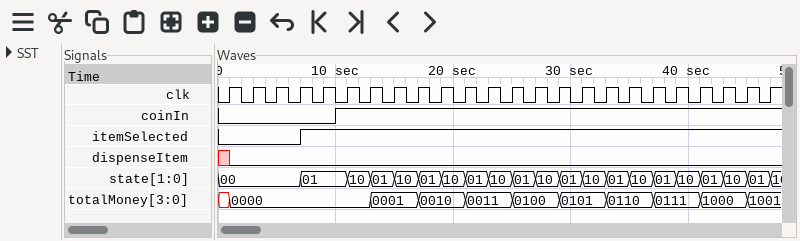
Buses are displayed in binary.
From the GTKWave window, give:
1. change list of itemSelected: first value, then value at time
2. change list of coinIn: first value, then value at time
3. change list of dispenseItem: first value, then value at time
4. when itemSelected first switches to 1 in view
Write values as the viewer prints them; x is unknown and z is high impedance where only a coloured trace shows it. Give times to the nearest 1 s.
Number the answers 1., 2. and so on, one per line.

1. 0, 1 at 7 s
2. 0, 1 at 10 s
3. x, 0 at 1 s
4. 7 s
